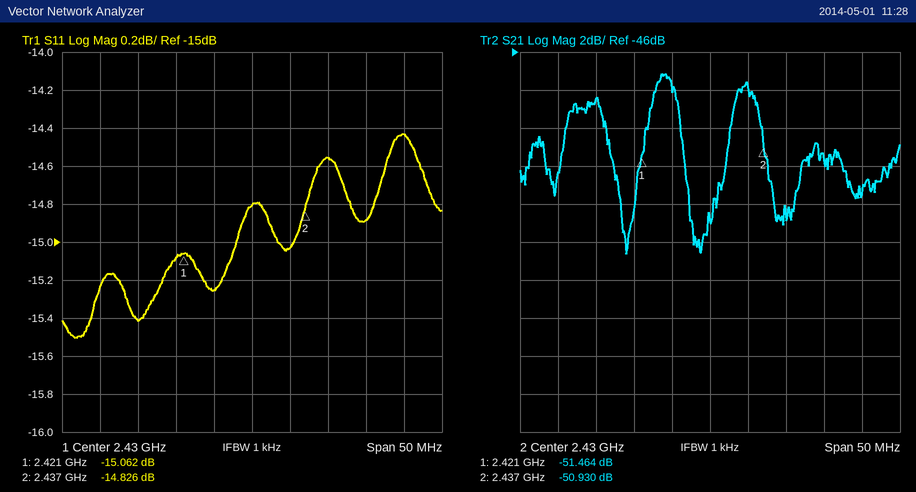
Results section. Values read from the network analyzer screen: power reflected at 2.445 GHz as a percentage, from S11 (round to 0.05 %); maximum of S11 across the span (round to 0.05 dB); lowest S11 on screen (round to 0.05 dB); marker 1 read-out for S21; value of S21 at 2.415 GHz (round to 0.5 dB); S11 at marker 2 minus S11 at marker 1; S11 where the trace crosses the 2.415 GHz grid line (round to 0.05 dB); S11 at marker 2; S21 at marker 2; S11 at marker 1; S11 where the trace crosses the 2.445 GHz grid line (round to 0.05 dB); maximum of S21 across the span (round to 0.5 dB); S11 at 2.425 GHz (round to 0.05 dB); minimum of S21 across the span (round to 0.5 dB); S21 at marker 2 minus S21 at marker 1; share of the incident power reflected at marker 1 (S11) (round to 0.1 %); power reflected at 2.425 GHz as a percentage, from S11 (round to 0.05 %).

3.25 %
-14.45 dB
-15.50 dB
-51.464 dB
-48.5 dB
0.236 dB
-15.40 dB
-14.826 dB
-50.930 dB
-15.062 dB
-14.90 dB
-47.0 dB
-15.25 dB
-56.5 dB
0.534 dB
3.1 %
3.00 %
